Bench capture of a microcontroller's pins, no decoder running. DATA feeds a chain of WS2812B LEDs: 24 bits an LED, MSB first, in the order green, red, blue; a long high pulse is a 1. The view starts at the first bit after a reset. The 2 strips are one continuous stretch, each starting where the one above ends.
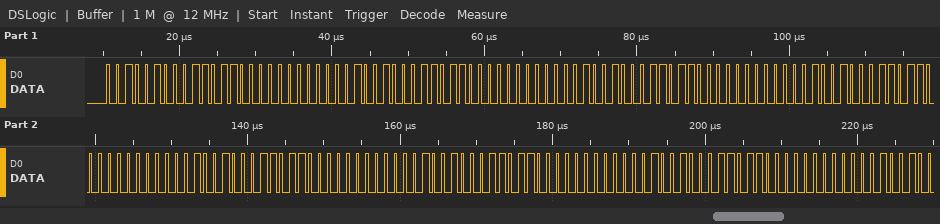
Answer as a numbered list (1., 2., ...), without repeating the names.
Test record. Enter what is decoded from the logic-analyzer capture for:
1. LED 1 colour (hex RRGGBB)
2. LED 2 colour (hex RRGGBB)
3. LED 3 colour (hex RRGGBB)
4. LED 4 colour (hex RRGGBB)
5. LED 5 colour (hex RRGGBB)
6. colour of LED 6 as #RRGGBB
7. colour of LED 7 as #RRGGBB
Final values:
1. #6C2400
2. #6C2400
3. #6C2400
4. #6C2400
5. #6C2400
6. #6C2400
7. #6C2400
